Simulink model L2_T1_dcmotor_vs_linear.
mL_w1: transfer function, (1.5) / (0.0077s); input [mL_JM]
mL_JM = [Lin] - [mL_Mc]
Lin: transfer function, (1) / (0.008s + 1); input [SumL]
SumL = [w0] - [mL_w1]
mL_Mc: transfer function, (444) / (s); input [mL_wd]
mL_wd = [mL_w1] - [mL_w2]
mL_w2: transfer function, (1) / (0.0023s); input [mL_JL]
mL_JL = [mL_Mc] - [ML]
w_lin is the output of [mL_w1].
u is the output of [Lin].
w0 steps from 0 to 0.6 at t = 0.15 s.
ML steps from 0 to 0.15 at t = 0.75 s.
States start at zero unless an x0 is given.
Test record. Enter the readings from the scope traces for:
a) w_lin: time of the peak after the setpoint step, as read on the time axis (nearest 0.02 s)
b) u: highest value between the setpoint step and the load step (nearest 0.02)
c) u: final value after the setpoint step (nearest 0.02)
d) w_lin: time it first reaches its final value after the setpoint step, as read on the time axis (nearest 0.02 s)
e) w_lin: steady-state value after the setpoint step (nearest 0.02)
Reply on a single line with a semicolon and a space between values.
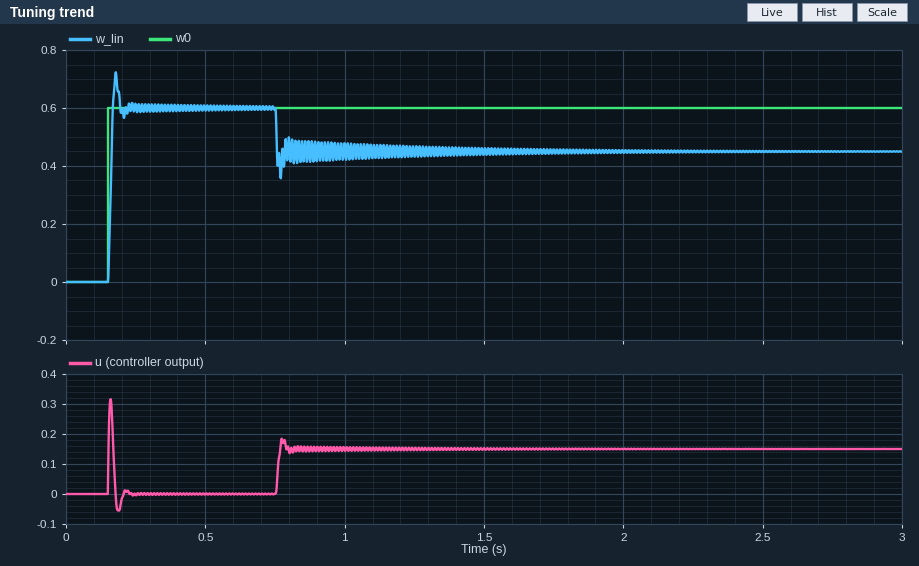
0.18 s; 0.32; 0.00; 0.16 s; 0.60
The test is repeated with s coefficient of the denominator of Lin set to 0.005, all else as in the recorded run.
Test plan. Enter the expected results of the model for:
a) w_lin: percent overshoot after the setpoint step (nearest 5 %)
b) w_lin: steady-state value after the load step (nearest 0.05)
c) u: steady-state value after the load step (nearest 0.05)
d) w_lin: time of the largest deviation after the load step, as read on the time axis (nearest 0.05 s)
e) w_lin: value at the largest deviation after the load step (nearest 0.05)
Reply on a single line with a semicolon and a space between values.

10 %; 0.45; 0.15; 0.75 s; 0.40
